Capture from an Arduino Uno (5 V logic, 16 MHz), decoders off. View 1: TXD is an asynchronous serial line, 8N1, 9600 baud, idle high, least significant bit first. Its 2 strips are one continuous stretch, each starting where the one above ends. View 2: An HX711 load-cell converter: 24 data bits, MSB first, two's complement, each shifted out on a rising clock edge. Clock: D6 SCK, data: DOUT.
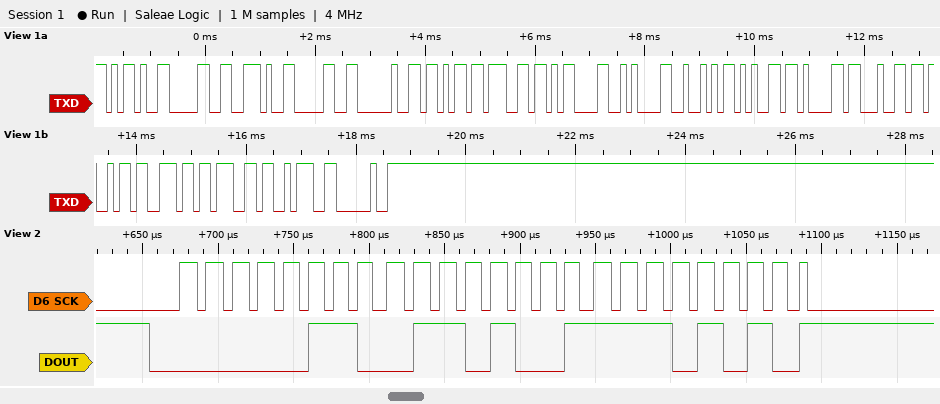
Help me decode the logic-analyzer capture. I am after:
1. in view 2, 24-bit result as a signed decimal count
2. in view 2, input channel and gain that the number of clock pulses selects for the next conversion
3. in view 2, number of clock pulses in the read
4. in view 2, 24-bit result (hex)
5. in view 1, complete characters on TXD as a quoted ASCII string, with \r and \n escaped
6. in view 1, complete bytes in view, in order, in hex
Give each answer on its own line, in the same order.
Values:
420330
channel A, gain 128
25
0x0669EA
"-0.0 kg\r\nReading: "
2D 30 2E 30 20 6B 67 0D 0A 52 65 61 64 69 6E 67 3A 20
